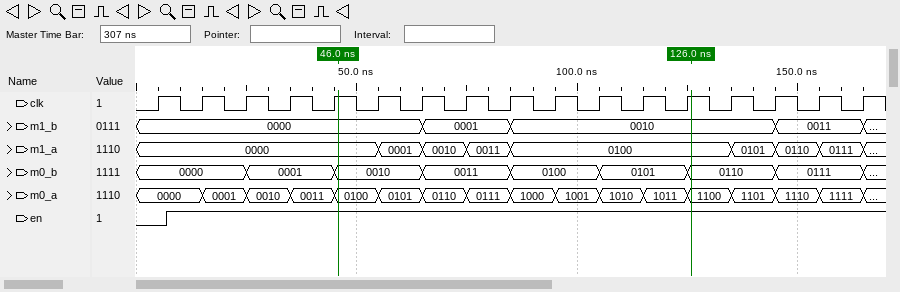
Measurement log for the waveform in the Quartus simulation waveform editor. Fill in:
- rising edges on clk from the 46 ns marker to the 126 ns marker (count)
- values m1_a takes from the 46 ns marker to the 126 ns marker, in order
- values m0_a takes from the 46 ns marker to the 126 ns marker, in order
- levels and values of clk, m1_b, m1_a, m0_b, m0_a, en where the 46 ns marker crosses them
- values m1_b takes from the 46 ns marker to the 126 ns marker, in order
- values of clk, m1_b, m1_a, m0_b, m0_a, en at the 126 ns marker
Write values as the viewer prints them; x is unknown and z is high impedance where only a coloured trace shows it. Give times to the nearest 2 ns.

8
0000, 0001, 0010, 0011, 0100
0100, 0101, 0110, 0111, 1000, 1001, 1010, 1011, 1100
clk=1, m1_b=0000, m1_a=0000, m0_b=0010, m0_a=0100, en=1
0000, 0001, 0010
clk=1, m1_b=0010, m1_a=0100, m0_b=0110, m0_a=1100, en=1
